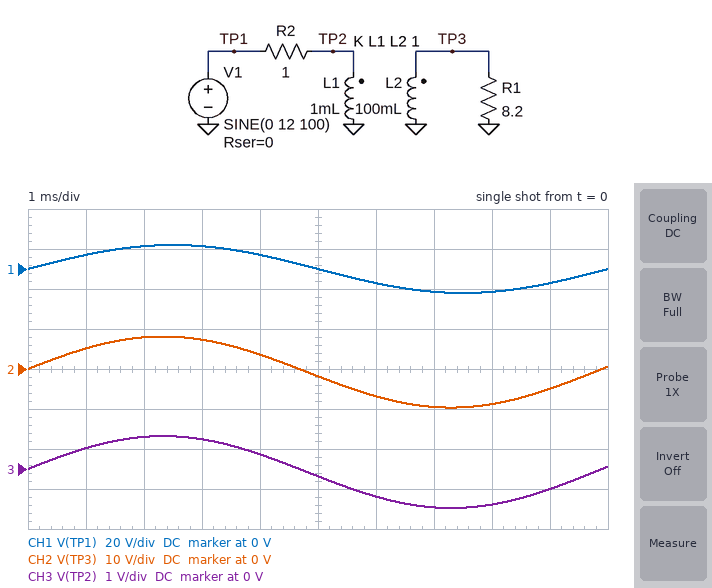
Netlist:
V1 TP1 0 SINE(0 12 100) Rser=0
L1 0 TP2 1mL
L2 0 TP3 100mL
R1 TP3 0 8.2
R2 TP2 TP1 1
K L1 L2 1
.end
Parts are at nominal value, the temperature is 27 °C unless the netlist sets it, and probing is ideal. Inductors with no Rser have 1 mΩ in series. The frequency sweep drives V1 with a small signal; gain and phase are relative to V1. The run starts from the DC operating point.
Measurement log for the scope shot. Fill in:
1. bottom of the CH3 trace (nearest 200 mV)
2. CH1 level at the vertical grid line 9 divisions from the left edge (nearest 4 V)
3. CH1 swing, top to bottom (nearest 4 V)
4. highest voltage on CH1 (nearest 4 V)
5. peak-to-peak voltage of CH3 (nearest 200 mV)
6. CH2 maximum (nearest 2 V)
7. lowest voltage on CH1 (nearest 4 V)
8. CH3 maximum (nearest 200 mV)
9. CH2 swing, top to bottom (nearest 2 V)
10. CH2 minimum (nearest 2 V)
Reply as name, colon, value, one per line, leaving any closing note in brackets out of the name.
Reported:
bottom of the CH3 trace: -1.0 V
CH1 level at the vertical grid line 9 divisions from the left edge: -8 V
CH1 swing, top to bottom: 24 V
highest voltage on CH1: 12 V
peak-to-peak voltage of CH3: 1.8 V
CH2 maximum: 8 V
lowest voltage on CH1: -12 V
CH3 maximum: 800 mV
CH2 swing, top to bottom: 18 V
CH2 minimum: -10 V
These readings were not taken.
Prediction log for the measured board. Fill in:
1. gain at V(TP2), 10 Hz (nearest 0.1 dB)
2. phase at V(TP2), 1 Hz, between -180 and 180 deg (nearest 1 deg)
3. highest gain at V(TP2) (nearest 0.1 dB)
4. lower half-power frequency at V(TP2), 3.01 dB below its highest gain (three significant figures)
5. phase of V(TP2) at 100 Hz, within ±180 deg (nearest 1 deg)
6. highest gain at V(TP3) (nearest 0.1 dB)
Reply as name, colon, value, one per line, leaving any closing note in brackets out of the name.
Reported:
gain at V(TP2), 10 Hz: -26.2 dB
phase at V(TP2), 1 Hz, between -180 and 180 deg: 76 deg
highest gain at V(TP2): -22.3 dB
lower half-power frequency at V(TP2), 3.01 dB below its highest gain: 12.1 Hz
phase of V(TP2) at 100 Hz, within ±180 deg: 7 deg
highest gain at V(TP3): -2.4 dB
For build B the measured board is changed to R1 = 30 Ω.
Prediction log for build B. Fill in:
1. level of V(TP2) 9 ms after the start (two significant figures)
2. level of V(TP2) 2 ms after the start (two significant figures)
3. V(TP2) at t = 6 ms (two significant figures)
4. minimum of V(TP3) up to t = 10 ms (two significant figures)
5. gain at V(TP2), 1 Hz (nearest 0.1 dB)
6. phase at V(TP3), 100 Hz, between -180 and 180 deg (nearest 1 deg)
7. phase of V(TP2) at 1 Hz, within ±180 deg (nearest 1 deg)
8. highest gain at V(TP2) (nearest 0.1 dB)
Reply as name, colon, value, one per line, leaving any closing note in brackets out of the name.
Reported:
level of V(TP2) 9 ms after the start: -830 mV
level of V(TP2) 2 ms after the start: 2.0 V
V(TP2) at t = 6 ms: -2.4 V
minimum of V(TP3) up to t = 10 ms: -28 V
gain at V(TP2), 1 Hz: -43.9 dB
phase at V(TP3), 100 Hz, between -180 and 180 deg: 20 deg
phase of V(TP2) at 1 Hz, within ±180 deg: 79 deg
highest gain at V(TP2): -12.7 dB
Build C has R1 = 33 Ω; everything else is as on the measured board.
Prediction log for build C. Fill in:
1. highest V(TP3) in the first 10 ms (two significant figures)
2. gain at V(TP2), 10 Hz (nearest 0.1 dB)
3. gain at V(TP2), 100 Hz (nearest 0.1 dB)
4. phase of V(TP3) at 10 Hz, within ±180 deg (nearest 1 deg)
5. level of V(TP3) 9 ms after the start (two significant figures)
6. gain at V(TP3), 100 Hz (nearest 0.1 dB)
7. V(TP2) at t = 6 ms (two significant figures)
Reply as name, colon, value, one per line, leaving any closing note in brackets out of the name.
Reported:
highest V(TP3) in the first 10 ms: 21 V
gain at V(TP2), 10 Hz: -24.3 dB
gain at V(TP2), 100 Hz: -12.7 dB
phase of V(TP3) at 10 Hz, within ±180 deg: 76 deg
level of V(TP3) 9 ms after the start: -8.0 V
gain at V(TP3), 100 Hz: 7.3 dB
V(TP2) at t = 6 ms: -2.6 V
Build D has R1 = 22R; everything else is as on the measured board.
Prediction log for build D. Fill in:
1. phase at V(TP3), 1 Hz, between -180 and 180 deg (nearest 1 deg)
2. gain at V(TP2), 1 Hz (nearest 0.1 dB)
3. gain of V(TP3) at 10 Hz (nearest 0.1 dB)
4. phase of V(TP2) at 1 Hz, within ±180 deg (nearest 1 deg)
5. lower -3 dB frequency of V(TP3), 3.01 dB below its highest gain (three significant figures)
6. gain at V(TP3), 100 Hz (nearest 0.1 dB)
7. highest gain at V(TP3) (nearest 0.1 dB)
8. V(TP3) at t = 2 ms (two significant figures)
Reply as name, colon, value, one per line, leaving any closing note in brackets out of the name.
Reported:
phase at V(TP3), 1 Hz, between -180 and 180 deg: 88 deg
gain at V(TP2), 1 Hz: -43.9 dB
gain of V(TP3) at 10 Hz: -4.5 dB
phase of V(TP2) at 1 Hz, within ±180 deg: 79 deg
lower -3 dB frequency of V(TP3), 3.01 dB below its highest gain: 28.7 Hz
gain at V(TP3), 100 Hz: 4.8 dB
highest gain at V(TP3): 5.1 dB
V(TP3) at t = 2 ms: 17 V
